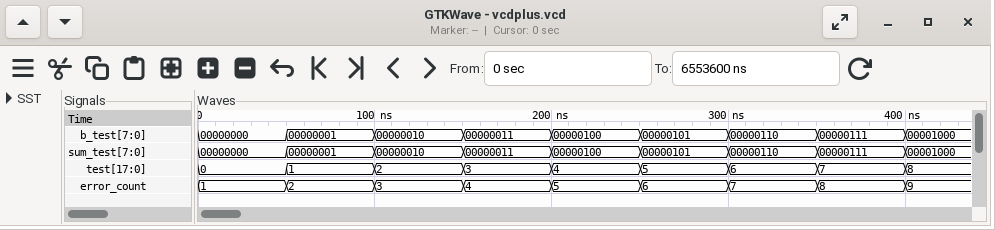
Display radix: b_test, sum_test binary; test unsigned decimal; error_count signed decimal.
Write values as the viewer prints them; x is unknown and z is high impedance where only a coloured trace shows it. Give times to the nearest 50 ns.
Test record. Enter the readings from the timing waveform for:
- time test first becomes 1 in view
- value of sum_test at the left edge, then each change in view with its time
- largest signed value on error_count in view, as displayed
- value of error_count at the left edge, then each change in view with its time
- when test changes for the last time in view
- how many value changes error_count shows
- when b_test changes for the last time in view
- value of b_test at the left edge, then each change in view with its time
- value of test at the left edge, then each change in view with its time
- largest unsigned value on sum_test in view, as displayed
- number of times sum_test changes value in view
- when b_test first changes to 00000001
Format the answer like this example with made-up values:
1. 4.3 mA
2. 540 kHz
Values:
1. 50 ns
2. 00000000, 00000001 at 50 ns, 00000010 at 100 ns, 00000011 at 150 ns, 00000100 at 200 ns, 00000101 at 250 ns, 00000110 at 300 ns, 00000111 at 350 ns, 00001000 at 400 ns
3. 9
4. 1, 2 at 50 ns, 3 at 100 ns, 4 at 150 ns, 5 at 200 ns, 6 at 250 ns, 7 at 300 ns, 8 at 350 ns, 9 at 400 ns
5. 400 ns
6. 8
7. 400 ns
8. 00000000, 00000001 at 50 ns, 00000010 at 100 ns, 00000011 at 150 ns, 00000100 at 200 ns, 00000101 at 250 ns, 00000110 at 300 ns, 00000111 at 350 ns, 00001000 at 400 ns
9. 0, 1 at 50 ns, 2 at 100 ns, 3 at 150 ns, 4 at 200 ns, 5 at 250 ns, 6 at 300 ns, 7 at 350 ns, 8 at 400 ns
10. 00001000
11. 8
12. 50 ns
